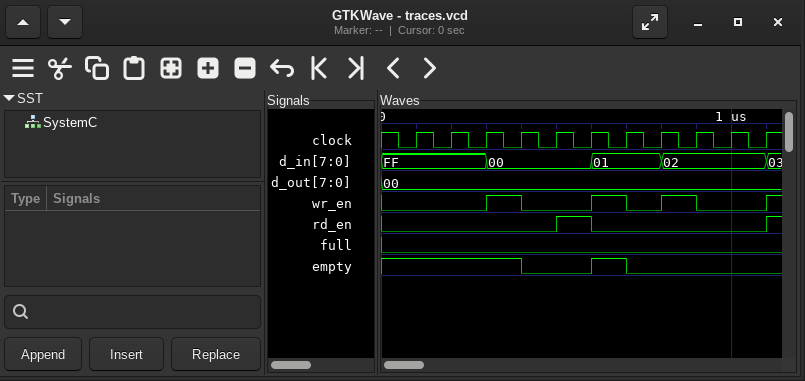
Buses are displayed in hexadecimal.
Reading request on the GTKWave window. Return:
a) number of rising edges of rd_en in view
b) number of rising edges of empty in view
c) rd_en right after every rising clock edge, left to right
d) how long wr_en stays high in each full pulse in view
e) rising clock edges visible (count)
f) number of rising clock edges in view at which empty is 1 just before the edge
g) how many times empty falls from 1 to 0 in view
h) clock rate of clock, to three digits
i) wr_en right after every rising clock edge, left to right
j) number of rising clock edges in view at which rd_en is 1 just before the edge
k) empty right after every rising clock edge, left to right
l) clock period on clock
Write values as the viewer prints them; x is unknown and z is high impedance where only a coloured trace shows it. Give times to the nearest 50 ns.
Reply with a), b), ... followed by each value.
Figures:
a) 2
b) 1
c) 0 0 0 0 1 0 0 0 0 0 1
d) 100 ns, 100 ns, 100 ns
e) 11
f) 5
g) 2
h) 10.0 MHz
i) 0 0 1 0 0 1 0 1 0 0 1
j) 1
k) 1 1 1 0 0 1 0 0 0 0 0
l) 100 ns
